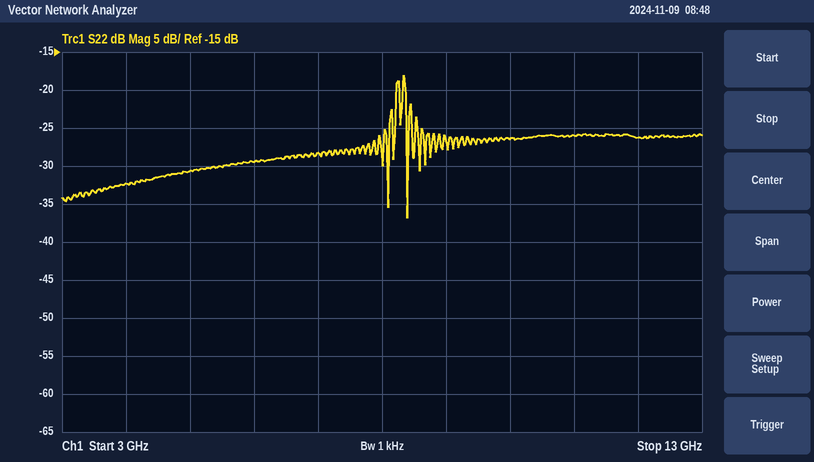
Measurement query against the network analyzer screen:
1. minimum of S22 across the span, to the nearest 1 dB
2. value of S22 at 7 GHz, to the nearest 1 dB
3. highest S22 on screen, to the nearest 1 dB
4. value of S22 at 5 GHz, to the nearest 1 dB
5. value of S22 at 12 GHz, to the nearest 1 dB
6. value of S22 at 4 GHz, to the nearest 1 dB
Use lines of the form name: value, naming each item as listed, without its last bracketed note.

minimum of S22 across the span, to the nearest 1 dB: -37 dB
value of S22 at 7 GHz, to the nearest 1 dB: -28 dB
highest S22 on screen, to the nearest 1 dB: -18 dB
value of S22 at 5 GHz, to the nearest 1 dB: -31 dB
value of S22 at 12 GHz, to the nearest 1 dB: -26 dB
value of S22 at 4 GHz, to the nearest 1 dB: -32 dB
